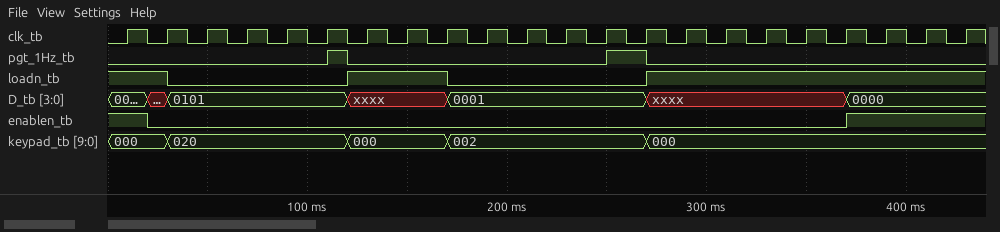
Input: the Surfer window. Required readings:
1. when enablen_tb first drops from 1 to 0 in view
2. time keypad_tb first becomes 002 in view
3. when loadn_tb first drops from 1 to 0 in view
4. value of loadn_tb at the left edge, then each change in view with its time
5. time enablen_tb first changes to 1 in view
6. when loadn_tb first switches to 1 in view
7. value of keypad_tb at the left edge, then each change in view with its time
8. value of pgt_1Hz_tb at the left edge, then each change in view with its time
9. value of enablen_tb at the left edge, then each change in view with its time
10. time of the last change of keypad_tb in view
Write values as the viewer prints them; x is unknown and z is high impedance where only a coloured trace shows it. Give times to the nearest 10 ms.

20 ms
170 ms
30 ms
1, 0 at 30 ms, 1 at 120 ms, 0 at 170 ms, 1 at 270 ms
370 ms
120 ms
000, 020 at 30 ms, 000 at 120 ms, 002 at 170 ms, 000 at 270 ms
0, 1 at 110 ms, 0 at 120 ms, 1 at 250 ms, 0 at 270 ms
1, 0 at 20 ms, 1 at 370 ms
270 ms
